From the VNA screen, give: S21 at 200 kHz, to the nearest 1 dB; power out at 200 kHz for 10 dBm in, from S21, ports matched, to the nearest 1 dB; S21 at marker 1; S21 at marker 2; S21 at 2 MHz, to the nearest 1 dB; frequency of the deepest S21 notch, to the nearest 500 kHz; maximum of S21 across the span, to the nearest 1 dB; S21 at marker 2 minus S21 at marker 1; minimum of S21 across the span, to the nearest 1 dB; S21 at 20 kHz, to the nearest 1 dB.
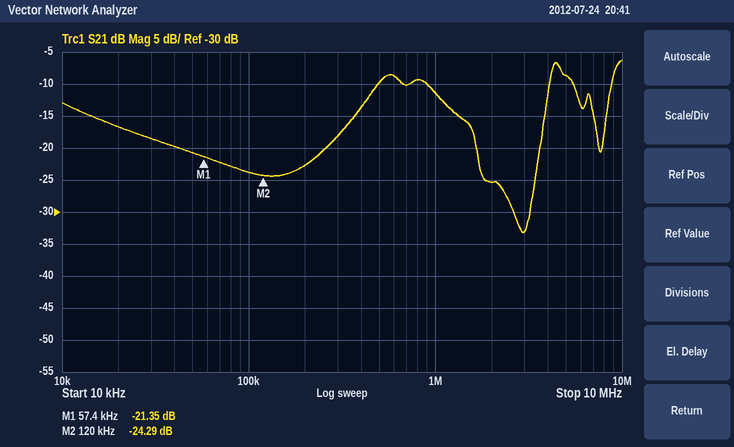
-23 dB
-13 dBm
-21.35 dB
-24.29 dB
-25 dB
3.0 MHz
-6 dB
-2.94 dB
-33 dB
-17 dB
